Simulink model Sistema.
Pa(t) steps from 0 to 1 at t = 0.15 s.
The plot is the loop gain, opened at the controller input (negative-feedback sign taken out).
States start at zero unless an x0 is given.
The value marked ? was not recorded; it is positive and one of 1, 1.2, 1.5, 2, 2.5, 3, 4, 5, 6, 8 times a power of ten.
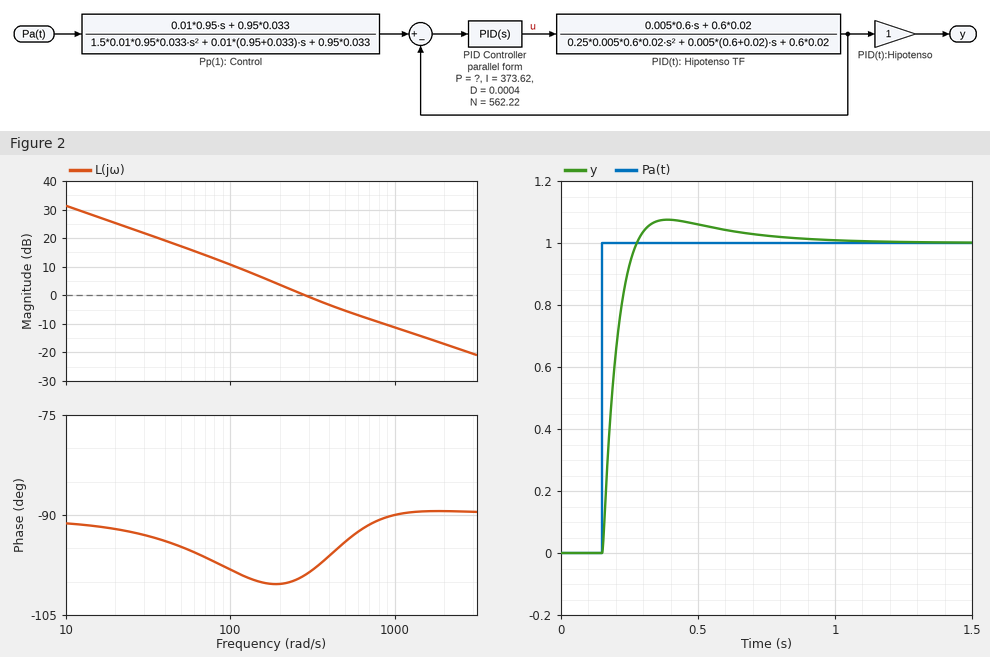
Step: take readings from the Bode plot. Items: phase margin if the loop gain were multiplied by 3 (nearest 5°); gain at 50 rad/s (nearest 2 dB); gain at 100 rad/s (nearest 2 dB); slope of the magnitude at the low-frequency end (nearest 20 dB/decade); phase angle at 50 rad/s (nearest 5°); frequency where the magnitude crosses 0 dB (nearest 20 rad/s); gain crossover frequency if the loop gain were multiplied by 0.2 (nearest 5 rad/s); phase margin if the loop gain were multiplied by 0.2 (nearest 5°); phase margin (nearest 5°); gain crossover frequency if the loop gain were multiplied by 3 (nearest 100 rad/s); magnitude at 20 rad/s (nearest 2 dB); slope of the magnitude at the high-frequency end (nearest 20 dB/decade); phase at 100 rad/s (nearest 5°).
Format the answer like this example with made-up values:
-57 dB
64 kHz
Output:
90°
18 dB
10 dB
-20 dB/decade
-95°
280 rad/s
70 rad/s
85°
80°
800 rad/s
26 dB
-20 dB/decade
-100°
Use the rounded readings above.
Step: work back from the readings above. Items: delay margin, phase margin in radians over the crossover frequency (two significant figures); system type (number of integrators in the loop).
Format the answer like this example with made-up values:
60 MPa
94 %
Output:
0.0050 s
1
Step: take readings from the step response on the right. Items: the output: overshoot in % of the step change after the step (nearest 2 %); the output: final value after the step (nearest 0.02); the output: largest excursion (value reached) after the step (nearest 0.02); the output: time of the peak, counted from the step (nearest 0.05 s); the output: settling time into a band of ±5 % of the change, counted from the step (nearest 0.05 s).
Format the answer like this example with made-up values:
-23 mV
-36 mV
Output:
8 %
1.00
1.08
0.25 s
0.40 s
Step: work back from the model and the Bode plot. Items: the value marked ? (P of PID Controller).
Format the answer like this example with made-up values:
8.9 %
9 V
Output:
1.2
